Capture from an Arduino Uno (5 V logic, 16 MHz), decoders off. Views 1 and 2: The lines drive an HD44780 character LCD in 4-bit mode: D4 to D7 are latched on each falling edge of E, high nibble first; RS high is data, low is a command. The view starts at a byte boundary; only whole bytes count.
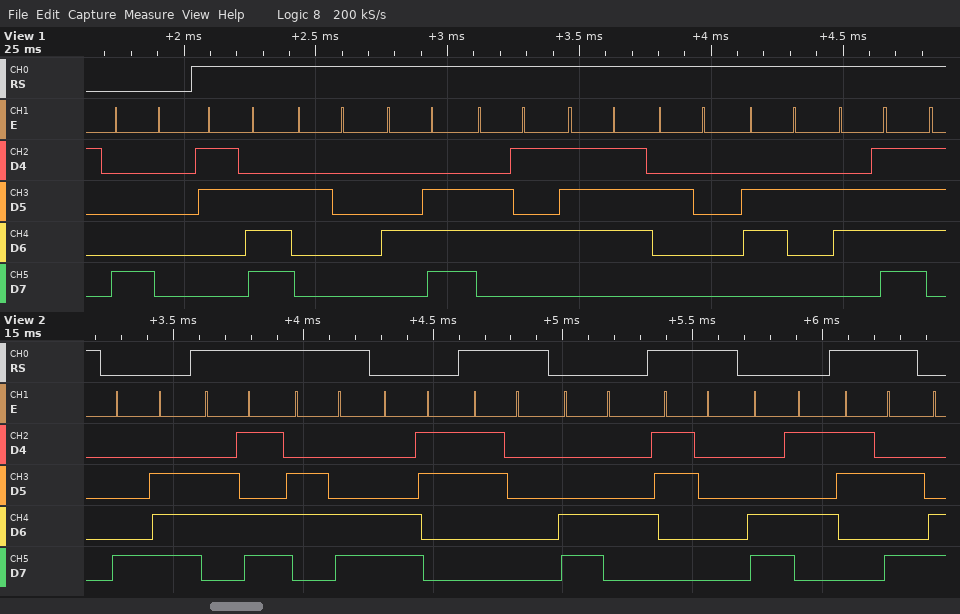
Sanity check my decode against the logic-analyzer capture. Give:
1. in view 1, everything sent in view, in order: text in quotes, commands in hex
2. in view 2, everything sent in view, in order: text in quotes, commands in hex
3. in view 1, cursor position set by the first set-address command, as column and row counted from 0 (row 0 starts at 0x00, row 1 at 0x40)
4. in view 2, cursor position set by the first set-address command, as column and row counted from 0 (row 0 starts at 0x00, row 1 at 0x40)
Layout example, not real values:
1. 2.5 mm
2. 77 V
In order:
1. 0x80 "> New bo"
2. 0x8E "ml" 0xC3 "0" 0xC4 "0" 0xC5 ":"
3. column 0, row 0
4. column 14, row 0
